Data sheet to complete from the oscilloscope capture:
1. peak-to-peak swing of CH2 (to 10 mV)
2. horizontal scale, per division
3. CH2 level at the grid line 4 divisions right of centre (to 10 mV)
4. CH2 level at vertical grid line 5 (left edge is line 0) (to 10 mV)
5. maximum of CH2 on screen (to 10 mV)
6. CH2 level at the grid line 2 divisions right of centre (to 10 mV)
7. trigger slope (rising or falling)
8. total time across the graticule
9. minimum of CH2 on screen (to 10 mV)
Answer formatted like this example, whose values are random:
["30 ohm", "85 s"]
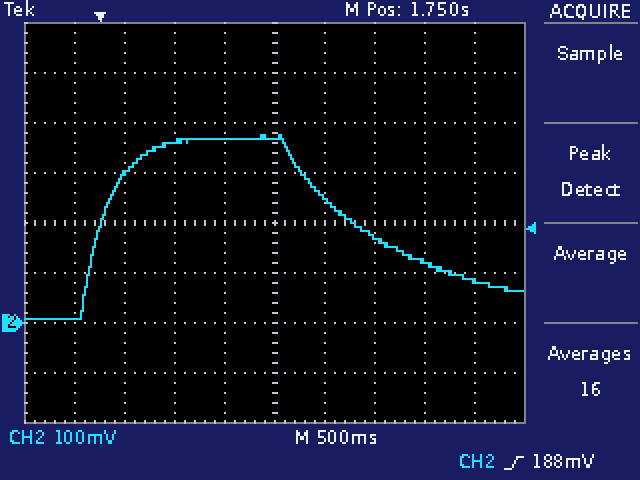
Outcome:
["370 mV", "500 ms", "80 mV", "370 mV", "380 mV", "170 mV", "rising", "5 s", "10 mV"]
